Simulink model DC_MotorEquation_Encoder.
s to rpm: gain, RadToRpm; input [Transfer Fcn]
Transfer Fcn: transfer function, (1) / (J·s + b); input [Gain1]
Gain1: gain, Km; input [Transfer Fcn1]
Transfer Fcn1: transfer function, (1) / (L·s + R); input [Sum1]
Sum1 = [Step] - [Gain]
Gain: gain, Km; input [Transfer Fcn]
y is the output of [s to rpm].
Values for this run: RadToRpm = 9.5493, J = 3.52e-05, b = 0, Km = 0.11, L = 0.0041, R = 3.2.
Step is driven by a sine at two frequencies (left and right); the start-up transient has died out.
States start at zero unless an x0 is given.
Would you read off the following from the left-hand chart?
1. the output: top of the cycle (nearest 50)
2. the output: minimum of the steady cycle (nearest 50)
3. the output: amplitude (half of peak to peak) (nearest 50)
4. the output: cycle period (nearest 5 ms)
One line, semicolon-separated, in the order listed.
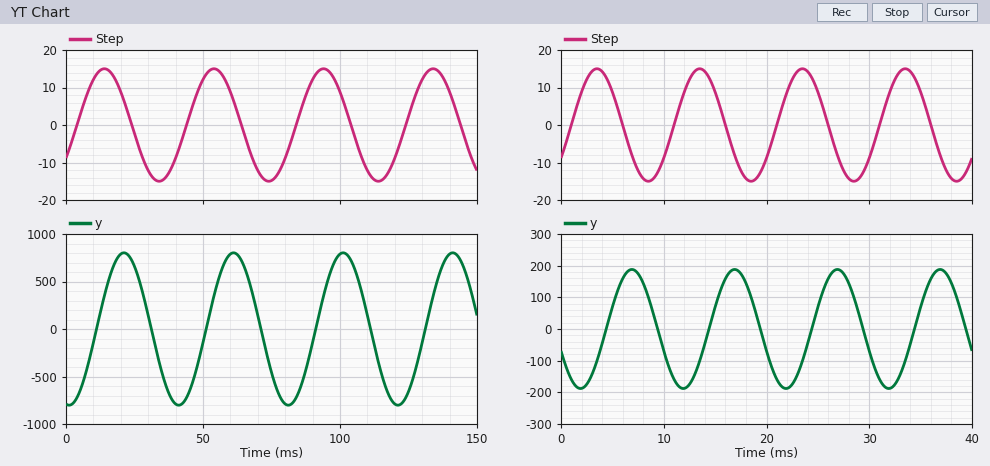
800; -800; 800; 40 ms
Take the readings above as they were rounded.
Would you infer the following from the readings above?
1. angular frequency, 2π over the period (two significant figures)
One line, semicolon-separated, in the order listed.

0.16 rad/ms
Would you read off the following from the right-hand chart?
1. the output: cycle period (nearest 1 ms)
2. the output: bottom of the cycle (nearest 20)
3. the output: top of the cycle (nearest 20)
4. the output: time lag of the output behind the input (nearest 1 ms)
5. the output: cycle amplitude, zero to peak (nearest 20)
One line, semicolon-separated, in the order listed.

10 ms; -180; 180; 3 ms; 180
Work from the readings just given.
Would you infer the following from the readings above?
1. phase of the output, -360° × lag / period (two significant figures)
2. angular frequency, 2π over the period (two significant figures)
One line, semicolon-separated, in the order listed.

-110°; 0.63 rad/ms
